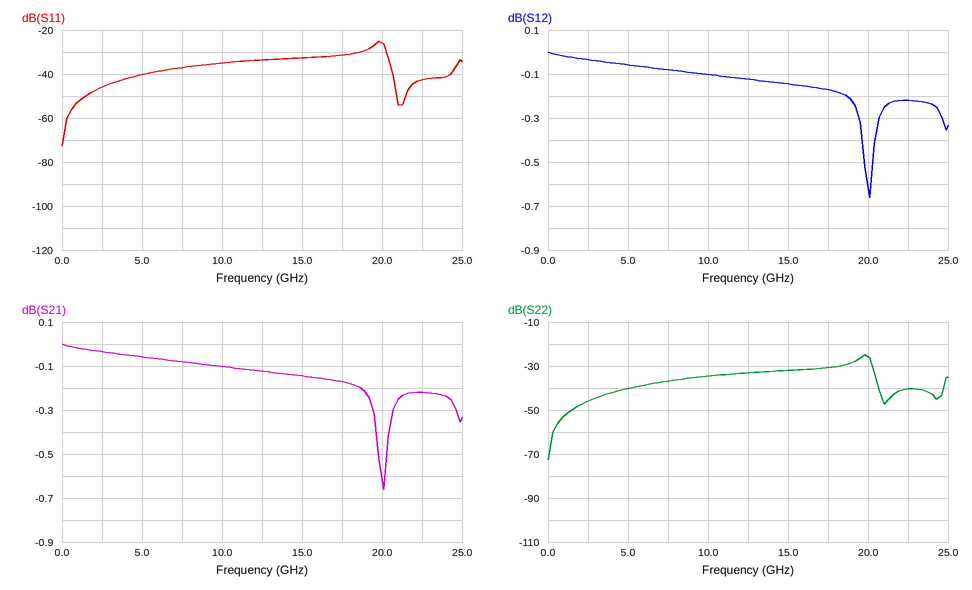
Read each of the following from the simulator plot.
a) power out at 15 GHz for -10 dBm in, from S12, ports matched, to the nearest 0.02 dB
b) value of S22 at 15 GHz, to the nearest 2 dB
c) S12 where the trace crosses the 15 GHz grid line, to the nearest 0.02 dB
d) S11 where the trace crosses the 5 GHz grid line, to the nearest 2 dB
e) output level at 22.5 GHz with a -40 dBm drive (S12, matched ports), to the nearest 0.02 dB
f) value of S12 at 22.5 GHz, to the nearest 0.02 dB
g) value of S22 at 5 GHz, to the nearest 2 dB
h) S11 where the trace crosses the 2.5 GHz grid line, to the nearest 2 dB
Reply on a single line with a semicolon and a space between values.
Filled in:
-10.14 dBm; -32 dB; -0.14 dB; -40 dB; -40.22 dBm; -0.22 dB; -40 dB; -46 dB
